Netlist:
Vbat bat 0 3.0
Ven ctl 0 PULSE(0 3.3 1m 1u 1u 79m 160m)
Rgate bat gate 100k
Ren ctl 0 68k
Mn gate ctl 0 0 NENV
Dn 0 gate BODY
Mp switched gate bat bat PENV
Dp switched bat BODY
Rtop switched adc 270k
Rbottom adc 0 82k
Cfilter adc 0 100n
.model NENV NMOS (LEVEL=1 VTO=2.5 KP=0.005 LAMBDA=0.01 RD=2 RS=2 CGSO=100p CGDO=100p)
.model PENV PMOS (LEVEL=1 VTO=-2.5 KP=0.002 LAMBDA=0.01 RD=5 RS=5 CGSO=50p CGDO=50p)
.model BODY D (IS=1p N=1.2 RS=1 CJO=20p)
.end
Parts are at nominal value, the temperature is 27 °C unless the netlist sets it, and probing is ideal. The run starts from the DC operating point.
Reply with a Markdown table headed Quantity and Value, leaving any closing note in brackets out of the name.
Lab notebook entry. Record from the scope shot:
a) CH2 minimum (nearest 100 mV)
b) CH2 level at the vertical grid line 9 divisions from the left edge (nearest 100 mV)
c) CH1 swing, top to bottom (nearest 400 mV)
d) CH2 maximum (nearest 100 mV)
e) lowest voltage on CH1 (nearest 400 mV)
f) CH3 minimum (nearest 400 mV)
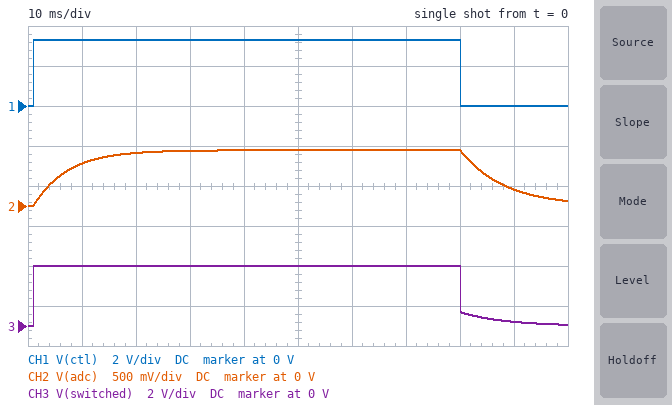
| Quantity | Value |
|---|---|
| CH2 minimum | 0 V |
| CH2 level at the vertical grid line 9 divisions from the left edge | 200 mV |
| CH1 swing, top to bottom | 3.2 V |
| CH2 maximum | 700 mV |
| lowest voltage on CH1 | 0 V |
| CH3 minimum | 0 V |
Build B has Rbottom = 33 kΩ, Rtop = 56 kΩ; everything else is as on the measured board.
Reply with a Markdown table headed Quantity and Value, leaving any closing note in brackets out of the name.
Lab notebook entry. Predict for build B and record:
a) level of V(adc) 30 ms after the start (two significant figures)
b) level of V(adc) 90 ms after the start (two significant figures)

| Quantity | Value |
|---|---|
| level of V(adc) 30 ms after the start | 1.1 V |
| level of V(adc) 90 ms after the start | 53 mV |
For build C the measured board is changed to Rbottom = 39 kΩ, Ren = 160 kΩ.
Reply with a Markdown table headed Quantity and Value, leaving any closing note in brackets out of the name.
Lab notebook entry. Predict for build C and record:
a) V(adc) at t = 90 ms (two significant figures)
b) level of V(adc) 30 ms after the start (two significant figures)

| Quantity | Value |
|---|---|
| V(adc) at t = 90 ms | 29 mV |
| level of V(adc) 30 ms after the start | 380 mV |
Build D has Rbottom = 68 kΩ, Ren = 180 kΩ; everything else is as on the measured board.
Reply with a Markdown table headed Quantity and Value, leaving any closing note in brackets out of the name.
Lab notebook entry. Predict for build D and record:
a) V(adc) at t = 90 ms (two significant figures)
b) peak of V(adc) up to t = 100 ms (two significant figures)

| Quantity | Value |
|---|---|
| V(adc) at t = 90 ms | 140 mV |
| peak of V(adc) up to t = 100 ms | 600 mV |
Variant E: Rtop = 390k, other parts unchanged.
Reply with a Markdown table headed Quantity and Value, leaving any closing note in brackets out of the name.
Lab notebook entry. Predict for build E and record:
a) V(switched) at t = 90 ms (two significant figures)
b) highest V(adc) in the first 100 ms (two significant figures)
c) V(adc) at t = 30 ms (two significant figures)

| Quantity | Value |
|---|---|
| V(switched) at t = 90 ms | 150 mV |
| highest V(adc) in the first 100 ms | 520 mV |
| V(adc) at t = 30 ms | 510 mV |
